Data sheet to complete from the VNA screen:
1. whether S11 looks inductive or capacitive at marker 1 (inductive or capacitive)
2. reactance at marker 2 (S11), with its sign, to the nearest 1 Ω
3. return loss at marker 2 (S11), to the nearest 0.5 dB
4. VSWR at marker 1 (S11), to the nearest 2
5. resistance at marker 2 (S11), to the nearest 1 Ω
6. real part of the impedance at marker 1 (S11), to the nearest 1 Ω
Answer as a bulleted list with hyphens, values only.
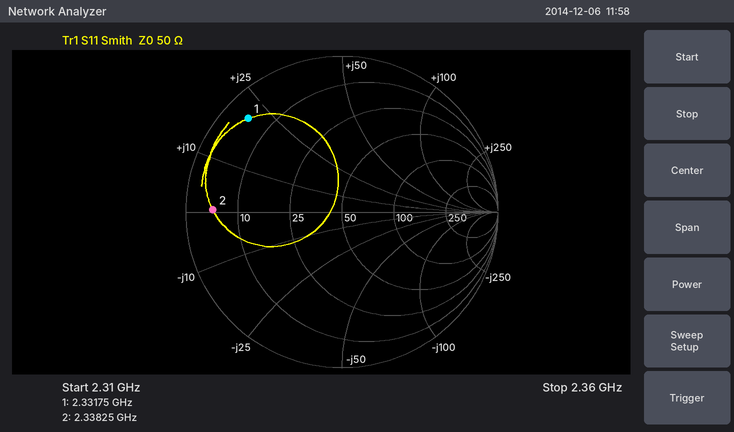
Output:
- inductive
- 0 Ω
- 1.5 dB
- 12
- 5 Ω
- 5 Ω
